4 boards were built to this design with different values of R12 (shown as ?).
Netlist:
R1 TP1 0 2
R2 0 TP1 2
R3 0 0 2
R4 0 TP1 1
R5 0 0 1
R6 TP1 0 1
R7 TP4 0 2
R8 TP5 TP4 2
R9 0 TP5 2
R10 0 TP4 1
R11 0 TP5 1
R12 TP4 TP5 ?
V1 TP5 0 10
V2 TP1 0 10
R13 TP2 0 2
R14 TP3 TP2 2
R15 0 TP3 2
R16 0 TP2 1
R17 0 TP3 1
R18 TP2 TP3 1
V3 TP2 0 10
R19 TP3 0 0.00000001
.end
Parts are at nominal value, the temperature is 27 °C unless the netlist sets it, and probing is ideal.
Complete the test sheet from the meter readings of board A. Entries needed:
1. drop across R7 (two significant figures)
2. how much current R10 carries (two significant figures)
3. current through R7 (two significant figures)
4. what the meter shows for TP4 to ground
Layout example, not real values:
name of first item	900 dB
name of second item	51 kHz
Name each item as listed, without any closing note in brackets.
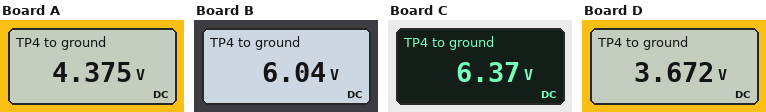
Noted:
drop across R7	4.4 V
how much current R10 carries	4.4 A
current through R7	2.2 A
what the meter shows for TP4 to ground	4.375 V
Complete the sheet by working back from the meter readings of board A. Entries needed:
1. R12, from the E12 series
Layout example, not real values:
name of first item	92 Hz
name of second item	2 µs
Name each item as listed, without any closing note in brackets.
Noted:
R12, from the E12 series	1.5 Ω
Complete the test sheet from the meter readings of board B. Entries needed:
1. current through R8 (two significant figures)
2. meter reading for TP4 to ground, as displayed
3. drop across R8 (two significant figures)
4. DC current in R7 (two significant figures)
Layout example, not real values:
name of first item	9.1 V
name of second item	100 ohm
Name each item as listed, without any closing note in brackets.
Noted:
current through R8	2.0 A
meter reading for TP4 to ground, as displayed	6.04 V
drop across R8	4.0 V
DC current in R7	3.0 A
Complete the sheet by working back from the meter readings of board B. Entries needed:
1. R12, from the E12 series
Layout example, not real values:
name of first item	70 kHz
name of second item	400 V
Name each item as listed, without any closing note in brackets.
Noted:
R12, from the E12 series	0.56 Ω
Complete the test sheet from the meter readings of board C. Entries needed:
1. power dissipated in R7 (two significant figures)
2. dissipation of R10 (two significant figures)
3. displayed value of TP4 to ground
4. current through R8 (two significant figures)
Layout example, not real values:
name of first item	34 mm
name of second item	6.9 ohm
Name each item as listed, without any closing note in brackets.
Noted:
power dissipated in R7	20 W
dissipation of R10	41 W
displayed value of TP4 to ground	6.37 V
current through R8	1.8 A
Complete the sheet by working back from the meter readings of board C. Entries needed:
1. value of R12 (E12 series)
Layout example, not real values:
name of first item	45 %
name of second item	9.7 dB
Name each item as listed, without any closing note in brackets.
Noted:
value of R12	0.47 Ω
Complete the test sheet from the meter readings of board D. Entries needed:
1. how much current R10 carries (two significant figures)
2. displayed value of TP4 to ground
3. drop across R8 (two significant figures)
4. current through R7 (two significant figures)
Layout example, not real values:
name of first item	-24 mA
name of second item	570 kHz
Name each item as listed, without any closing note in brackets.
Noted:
how much current R10 carries	3.7 A
displayed value of TP4 to ground	3.672 V
drop across R8	6.3 V
current through R7	1.8 A
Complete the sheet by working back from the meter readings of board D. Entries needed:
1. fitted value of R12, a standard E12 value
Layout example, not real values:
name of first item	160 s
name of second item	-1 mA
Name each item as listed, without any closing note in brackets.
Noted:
fitted value of R12, a standard E12 value	2.7 Ω
